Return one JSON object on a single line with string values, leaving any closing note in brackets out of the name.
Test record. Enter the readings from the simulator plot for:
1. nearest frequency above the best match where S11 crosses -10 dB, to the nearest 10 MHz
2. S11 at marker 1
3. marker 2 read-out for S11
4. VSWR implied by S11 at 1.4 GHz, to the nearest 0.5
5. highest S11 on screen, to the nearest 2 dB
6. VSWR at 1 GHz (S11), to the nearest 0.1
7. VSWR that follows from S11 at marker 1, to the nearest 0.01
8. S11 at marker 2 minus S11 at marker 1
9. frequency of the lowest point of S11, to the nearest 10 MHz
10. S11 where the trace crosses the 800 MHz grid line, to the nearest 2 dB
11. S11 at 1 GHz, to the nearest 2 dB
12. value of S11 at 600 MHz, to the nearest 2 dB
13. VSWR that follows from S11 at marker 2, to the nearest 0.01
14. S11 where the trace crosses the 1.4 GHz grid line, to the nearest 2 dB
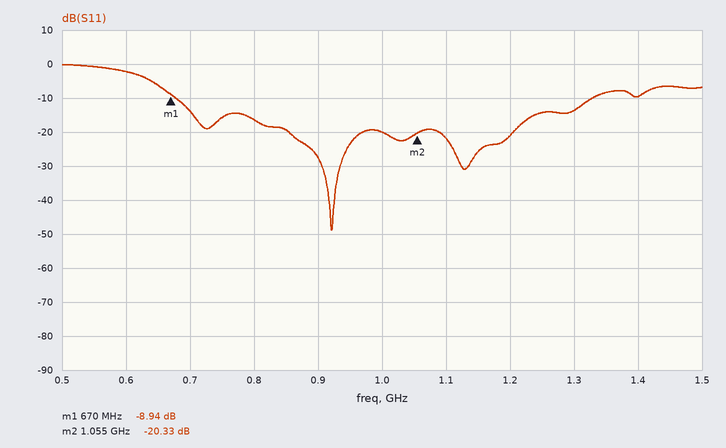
{"nearest frequency above the best match where S11 crosses -10 dB, to the nearest 10 MHz": "1.33 GHz", "S11 at marker 1": "-8.94 dB", "marker 2 read-out for S11": "-20.33 dB", "VSWR implied by S11 at 1.4 GHz, to the nearest 0.5": "2.0", "highest S11 on screen, to the nearest 2 dB": "0 dB", "VSWR at 1 GHz (S11), to the nearest 0.1": "1.2", "VSWR that follows from S11 at marker 1, to the nearest 0.01": "2.11", "S11 at marker 2 minus S11 at marker 1": "-11.39 dB", "frequency of the lowest point of S11, to the nearest 10 MHz": "920 MHz", "S11 where the trace crosses the 800 MHz grid line, to the nearest 2 dB": "-16 dB", "S11 at 1 GHz, to the nearest 2 dB": "-20 dB", "value of S11 at 600 MHz, to the nearest 2 dB": "-2 dB", "VSWR that follows from S11 at marker 2, to the nearest 0.01": "1.21", "S11 where the trace crosses the 1.4 GHz grid line, to the nearest 2 dB": "-10 dB"}
